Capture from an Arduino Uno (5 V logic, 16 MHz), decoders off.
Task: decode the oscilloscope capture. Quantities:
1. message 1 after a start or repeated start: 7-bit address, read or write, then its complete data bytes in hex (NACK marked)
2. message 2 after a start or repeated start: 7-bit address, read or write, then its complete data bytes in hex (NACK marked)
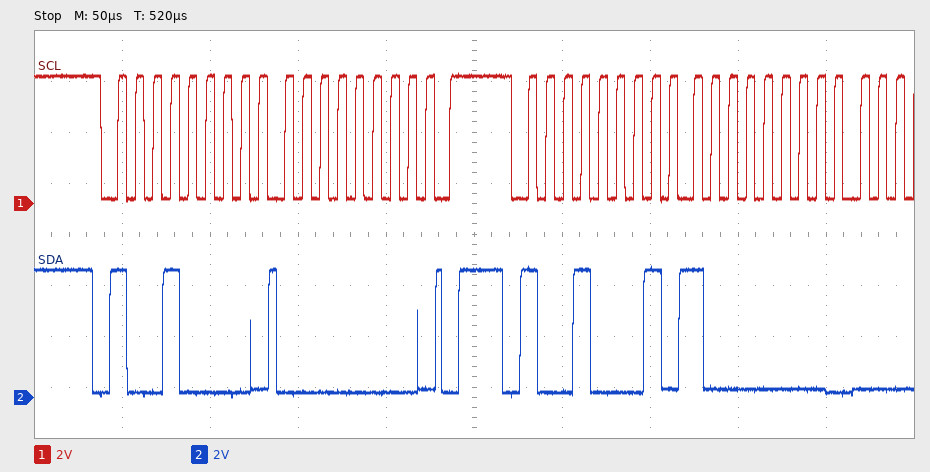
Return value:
0x48 write: 00
0x48 read: 80
